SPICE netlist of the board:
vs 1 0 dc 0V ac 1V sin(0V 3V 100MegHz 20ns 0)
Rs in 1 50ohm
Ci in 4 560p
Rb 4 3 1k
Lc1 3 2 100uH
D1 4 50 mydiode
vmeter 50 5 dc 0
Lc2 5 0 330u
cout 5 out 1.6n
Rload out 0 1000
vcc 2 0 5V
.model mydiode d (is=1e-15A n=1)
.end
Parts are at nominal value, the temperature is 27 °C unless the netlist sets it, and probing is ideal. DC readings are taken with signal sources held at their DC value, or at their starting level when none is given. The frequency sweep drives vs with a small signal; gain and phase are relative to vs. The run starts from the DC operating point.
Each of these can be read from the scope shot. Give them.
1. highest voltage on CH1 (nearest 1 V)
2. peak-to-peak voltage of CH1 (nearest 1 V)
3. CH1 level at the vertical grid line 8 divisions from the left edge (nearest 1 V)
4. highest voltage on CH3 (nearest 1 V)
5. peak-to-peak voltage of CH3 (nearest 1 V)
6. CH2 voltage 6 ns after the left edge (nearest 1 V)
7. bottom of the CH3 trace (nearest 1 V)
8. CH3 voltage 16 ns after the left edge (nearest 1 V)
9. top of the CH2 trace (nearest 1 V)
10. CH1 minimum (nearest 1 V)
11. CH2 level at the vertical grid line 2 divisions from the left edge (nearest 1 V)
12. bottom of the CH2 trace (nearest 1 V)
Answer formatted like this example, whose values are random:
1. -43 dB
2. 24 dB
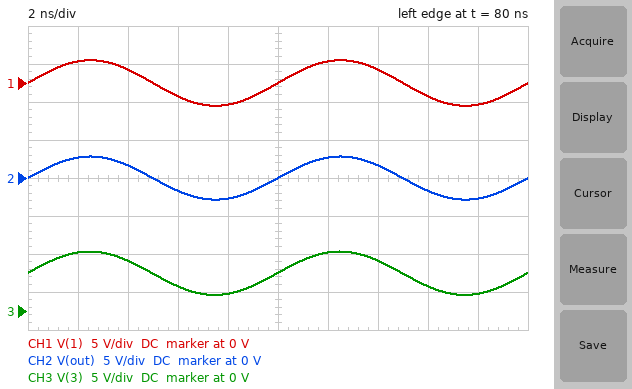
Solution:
1. 3 V
2. 6 V
3. -2 V
4. 8 V
5. 6 V
6. -2 V
7. 2 V
8. 3 V
9. 3 V
10. -3 V
11. 2 V
12. -3 V
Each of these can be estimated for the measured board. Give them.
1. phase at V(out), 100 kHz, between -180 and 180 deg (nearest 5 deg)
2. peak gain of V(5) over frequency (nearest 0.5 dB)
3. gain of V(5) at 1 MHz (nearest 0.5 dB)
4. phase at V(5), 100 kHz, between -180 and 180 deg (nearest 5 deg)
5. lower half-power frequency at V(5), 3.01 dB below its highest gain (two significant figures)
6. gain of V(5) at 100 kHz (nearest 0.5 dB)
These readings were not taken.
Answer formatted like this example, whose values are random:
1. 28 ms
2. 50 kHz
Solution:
1. -155 deg
2. 0 dB
3. 0 dB
4. 160 deg
5. 410 kHz
6. -22.0 dB
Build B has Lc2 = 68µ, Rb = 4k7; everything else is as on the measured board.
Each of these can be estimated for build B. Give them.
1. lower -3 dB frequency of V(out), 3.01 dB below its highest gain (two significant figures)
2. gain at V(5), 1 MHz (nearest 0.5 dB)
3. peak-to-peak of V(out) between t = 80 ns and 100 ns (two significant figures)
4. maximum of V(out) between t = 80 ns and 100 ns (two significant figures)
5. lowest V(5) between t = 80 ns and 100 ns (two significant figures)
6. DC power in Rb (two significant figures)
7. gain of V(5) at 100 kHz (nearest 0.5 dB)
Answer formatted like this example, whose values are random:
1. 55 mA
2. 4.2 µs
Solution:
1. 650 kHz
2. 3.5 dB
3. 4.1 V
4. 2.7 V
5. -1.4 V
6. 3.9 mW
7. -36.0 dB
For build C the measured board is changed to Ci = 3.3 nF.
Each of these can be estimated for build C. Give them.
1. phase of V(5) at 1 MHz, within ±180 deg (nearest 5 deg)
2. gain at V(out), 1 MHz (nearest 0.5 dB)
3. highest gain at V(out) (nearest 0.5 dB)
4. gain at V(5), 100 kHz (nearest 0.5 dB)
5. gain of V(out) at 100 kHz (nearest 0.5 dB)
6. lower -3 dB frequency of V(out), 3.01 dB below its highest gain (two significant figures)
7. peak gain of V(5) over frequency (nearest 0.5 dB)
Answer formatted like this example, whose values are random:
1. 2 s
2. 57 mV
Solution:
1. 5 deg
2. -0.5 dB
3. 1.5 dB
4. -3.0 dB
5. -6.0 dB
6. 120 kHz
7. 3.0 dB
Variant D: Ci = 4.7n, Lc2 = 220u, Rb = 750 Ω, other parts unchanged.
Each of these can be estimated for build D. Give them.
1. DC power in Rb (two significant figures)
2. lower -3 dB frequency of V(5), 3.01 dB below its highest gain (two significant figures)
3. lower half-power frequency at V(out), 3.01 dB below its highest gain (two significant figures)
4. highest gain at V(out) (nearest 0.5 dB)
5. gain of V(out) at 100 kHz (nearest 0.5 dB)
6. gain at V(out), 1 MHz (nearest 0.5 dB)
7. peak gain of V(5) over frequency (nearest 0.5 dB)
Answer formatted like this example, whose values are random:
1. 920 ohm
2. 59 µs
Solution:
1. 24 mW
2. 120 kHz
3. 130 kHz
4. 2.0 dB
5. -7.0 dB
6. -0.5 dB
7. 3.0 dB
